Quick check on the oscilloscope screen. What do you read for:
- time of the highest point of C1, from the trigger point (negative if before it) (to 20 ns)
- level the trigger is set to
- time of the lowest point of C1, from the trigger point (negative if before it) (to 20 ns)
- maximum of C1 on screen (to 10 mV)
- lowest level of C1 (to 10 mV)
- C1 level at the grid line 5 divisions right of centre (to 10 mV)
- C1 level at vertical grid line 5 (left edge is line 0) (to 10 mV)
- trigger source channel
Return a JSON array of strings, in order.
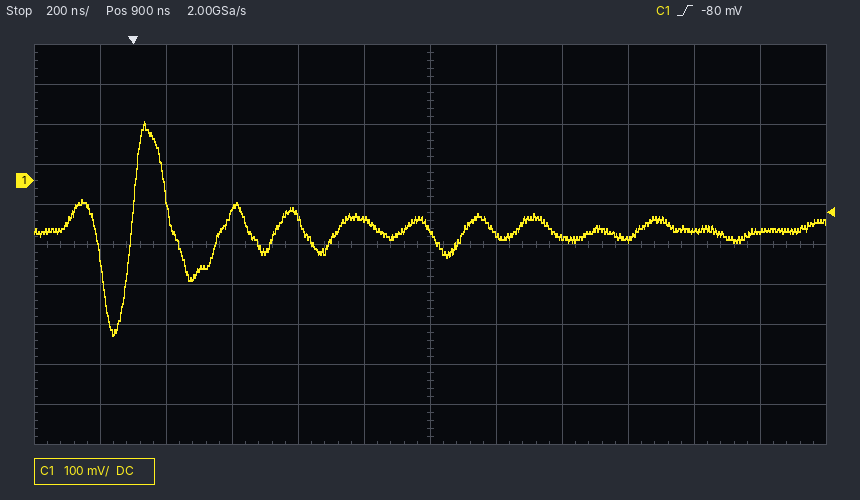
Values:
["+40 ns", "-80 mV", "-60 ns", "150 mV", "-390 mV", "-130 mV", "-100 mV", "C1"]
